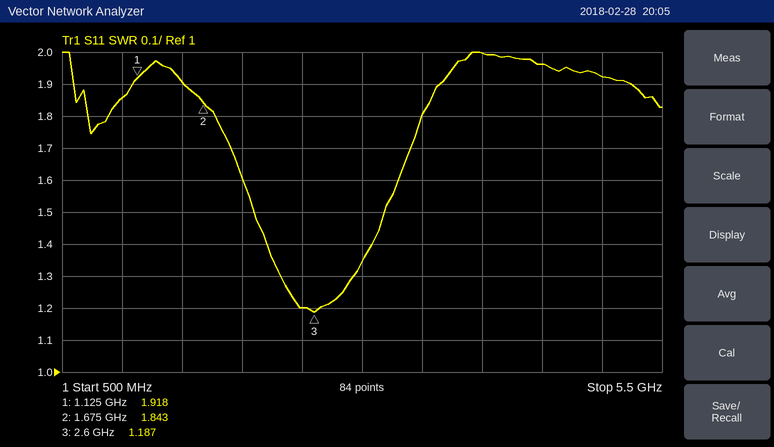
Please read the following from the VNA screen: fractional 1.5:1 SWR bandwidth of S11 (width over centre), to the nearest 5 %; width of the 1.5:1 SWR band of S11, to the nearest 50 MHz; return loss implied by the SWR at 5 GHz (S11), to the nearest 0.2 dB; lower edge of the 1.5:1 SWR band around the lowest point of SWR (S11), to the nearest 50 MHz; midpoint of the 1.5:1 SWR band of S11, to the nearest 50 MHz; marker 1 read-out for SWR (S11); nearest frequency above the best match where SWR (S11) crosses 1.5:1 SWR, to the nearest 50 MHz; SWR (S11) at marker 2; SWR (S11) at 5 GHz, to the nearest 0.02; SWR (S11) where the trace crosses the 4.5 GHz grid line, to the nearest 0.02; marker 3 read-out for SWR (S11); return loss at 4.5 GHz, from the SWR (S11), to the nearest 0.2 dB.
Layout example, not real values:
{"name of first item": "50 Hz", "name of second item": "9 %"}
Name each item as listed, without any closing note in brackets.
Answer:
{"fractional 1.5:1 SWR bandwidth of S11 (width over centre), to the nearest 5 %": "40 %", "width of the 1.5:1 SWR band of S11, to the nearest 50 MHz": "1.10 GHz", "return loss implied by the SWR at 5 GHz (S11), to the nearest 0.2 dB": "10.0 dB", "lower edge of the 1.5:1 SWR band around the lowest point of SWR (S11), to the nearest 50 MHz": "2.10 GHz", "midpoint of the 1.5:1 SWR band of S11, to the nearest 50 MHz": "2.65 GHz", "marker 1 read-out for SWR": "1.918", "nearest frequency above the best match where SWR (S11) crosses 1.5:1 SWR, to the nearest 50 MHz": "3.20 GHz", "SWR (S11) at marker 2": "1.843", "SWR (S11) at 5 GHz, to the nearest 0.02": "1.92", "SWR (S11) where the trace crosses the 4.5 GHz grid line, to the nearest 0.02": "1.96", "marker 3 read-out for SWR": "1.187", "return loss at 4.5 GHz, from the SWR (S11), to the nearest 0.2 dB": "9.8 dB"}
